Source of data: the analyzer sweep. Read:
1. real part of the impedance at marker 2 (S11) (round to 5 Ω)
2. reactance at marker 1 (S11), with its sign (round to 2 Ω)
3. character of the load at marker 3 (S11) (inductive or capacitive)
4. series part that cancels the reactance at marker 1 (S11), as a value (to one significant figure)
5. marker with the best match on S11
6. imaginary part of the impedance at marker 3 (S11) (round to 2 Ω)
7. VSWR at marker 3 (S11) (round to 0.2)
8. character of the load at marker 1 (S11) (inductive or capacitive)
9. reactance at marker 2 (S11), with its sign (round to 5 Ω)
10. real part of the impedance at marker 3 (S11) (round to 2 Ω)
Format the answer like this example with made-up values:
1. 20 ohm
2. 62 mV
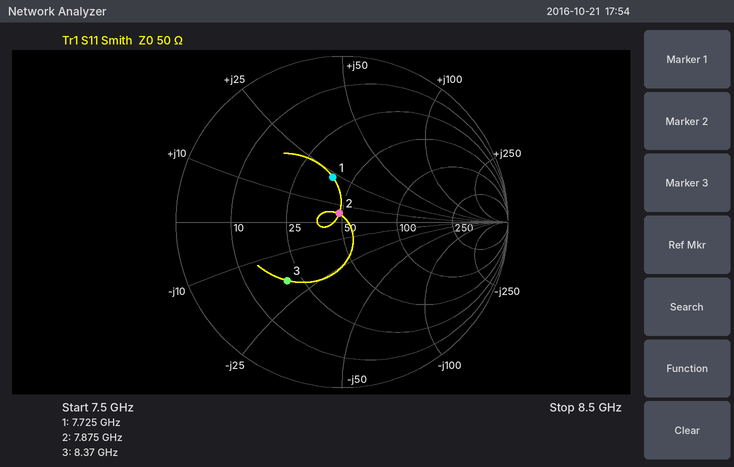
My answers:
1. 50 Ω
2. +22 Ω
3. capacitive
4. 900 fF
5. marker 2
6. -18 Ω
7. 2.8
8. inductive
9. +5 Ω
10. 20 Ω
